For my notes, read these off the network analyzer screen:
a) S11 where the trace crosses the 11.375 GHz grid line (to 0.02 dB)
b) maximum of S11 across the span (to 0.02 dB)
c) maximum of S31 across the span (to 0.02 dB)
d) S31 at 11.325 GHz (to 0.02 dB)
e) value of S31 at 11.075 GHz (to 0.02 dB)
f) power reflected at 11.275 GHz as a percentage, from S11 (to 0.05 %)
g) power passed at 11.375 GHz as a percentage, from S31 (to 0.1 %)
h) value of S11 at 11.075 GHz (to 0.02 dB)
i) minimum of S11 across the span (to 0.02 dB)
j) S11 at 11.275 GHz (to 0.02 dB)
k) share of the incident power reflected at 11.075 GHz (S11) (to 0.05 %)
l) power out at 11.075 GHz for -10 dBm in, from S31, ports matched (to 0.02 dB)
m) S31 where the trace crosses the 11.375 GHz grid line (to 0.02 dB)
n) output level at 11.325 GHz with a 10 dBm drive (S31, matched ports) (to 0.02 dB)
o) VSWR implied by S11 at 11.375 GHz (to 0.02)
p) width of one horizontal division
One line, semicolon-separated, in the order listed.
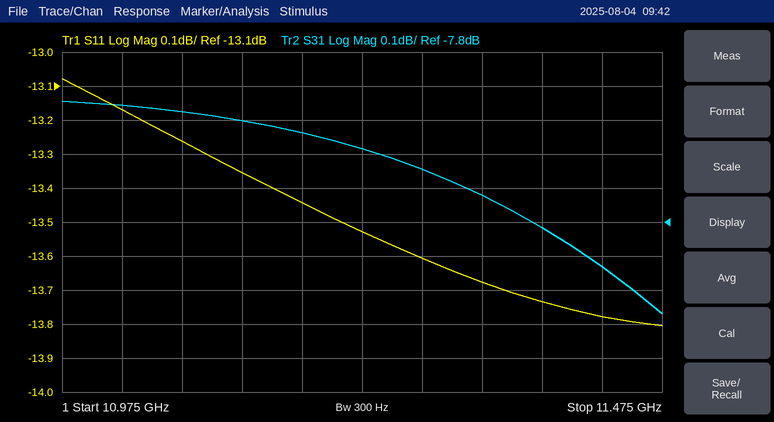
-13.74 dB; -13.08 dB; -7.44 dB; -7.72 dB; -7.48 dB; 4.35 %; 16.5 %; -13.26 dB; -13.80 dB; -13.60 dB; 4.70 %; -17.48 dBm; -7.82 dB; 2.28 dBm; 1.52; 50 MHz
